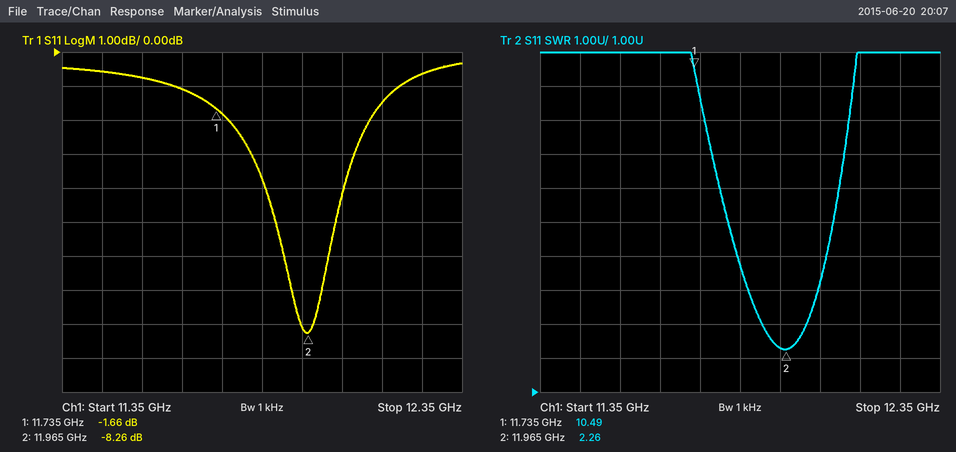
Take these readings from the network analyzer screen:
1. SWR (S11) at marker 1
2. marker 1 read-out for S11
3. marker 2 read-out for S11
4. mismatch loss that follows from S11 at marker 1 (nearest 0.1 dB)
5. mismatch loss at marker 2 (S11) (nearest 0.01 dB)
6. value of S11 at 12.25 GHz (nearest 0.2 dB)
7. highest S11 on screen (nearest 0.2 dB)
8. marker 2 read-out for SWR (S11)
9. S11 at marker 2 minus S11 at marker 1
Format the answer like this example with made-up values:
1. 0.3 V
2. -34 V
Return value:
1. 10.49
2. -1.66 dB
3. -8.26 dB
4. 5.0 dB
5. 0.70 dB
6. -0.6 dB
7. -0.4 dB
8. 2.26
9. -6.60 dB
